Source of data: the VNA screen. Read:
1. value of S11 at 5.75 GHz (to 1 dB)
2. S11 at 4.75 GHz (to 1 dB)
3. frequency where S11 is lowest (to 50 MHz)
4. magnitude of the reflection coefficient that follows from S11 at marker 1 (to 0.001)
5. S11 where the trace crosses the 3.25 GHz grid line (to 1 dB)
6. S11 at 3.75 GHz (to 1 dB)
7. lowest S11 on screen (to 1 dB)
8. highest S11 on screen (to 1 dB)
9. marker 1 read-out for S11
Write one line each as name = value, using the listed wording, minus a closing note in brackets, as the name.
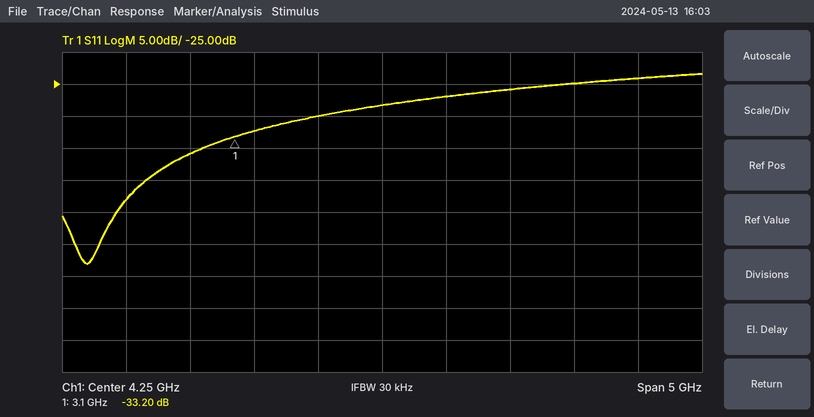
value of S11 at 5.75 GHz = -25 dB
S11 at 4.75 GHz = -27 dB
frequency where S11 is lowest = 1.95 GHz
magnitude of the reflection coefficient that follows from S11 at marker 1 = 0.022
S11 where the trace crosses the 3.25 GHz grid line = -32 dB
S11 at 3.75 GHz = -30 dB
lowest S11 on screen = -53 dB
highest S11 on screen = -23 dB
marker 1 read-out for S11 = -33.20 dB
